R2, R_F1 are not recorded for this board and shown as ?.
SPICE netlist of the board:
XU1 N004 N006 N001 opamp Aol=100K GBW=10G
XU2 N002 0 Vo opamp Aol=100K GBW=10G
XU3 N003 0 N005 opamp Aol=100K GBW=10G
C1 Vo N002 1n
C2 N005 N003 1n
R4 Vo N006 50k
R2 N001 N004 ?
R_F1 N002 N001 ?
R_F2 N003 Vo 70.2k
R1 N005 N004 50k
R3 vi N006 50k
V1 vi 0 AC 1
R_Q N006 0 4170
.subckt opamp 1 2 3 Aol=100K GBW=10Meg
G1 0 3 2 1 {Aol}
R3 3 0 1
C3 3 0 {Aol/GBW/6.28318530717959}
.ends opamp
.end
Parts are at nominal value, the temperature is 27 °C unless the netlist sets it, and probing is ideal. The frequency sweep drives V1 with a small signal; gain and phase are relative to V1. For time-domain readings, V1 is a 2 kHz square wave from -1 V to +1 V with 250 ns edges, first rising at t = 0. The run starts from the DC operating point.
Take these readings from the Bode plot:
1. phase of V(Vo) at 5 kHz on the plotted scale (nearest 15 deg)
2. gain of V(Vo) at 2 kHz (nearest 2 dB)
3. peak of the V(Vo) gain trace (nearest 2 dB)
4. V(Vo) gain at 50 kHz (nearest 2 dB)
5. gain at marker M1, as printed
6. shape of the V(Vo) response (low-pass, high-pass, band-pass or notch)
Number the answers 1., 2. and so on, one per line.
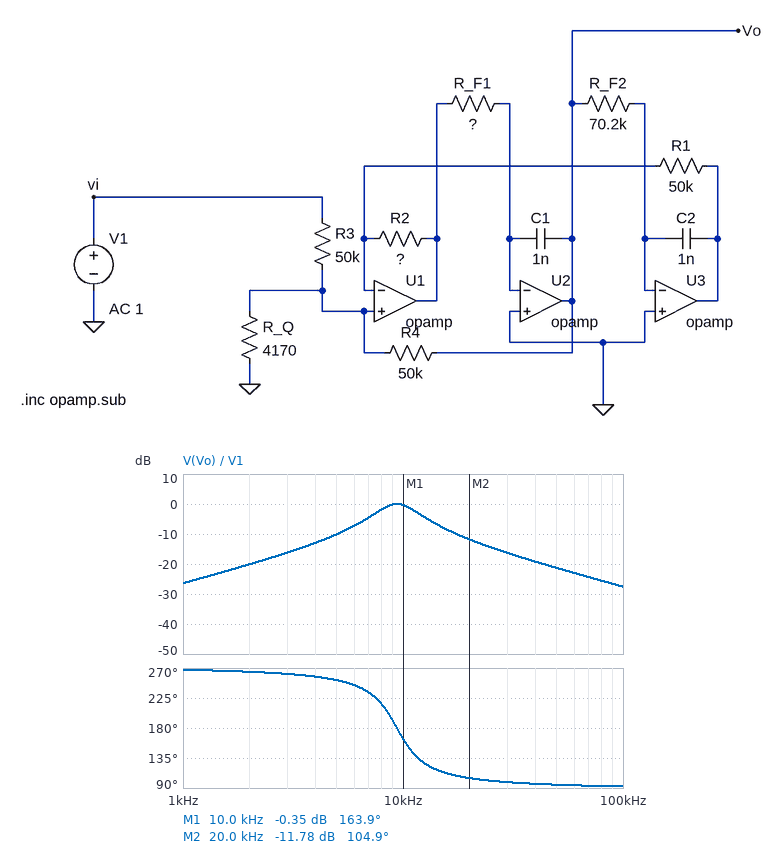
1. 255 deg
2. -20 dB
3. 0 dB
4. -22 dB
5. -0.35 dB
6. band-pass
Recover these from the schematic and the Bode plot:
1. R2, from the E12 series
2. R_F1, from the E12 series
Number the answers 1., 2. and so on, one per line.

1. 100 kΩ
2. 8.2 kΩ
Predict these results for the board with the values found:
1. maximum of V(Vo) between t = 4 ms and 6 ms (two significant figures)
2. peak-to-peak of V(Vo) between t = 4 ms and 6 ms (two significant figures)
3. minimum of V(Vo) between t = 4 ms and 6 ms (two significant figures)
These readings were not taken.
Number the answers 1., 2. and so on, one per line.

1. 650 mV
2. 1.3 V
3. -650 mV
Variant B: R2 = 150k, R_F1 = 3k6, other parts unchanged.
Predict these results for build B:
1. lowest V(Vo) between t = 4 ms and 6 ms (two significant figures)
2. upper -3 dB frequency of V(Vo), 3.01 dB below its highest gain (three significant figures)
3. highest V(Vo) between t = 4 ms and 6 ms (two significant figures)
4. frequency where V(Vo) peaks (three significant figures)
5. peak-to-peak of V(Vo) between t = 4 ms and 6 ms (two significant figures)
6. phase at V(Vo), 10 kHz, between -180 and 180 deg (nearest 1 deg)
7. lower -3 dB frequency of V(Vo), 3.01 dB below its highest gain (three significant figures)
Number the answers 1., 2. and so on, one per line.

1. -910 mV
2. 24.8 kHz
3. 910 mV
4. 17.3 kHz
5. 1.8 V
6. -122 deg
7. 12.1 kHz
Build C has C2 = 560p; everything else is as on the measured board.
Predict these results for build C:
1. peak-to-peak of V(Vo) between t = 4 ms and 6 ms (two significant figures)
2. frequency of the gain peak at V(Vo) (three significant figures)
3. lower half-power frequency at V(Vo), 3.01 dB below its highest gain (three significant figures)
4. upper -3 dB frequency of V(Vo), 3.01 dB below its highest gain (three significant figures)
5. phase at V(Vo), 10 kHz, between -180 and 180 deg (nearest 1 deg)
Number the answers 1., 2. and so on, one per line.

1. 1.0 V
2. 12.5 kHz
3. 10.6 kHz
4. 14.8 kHz
5. -126 deg
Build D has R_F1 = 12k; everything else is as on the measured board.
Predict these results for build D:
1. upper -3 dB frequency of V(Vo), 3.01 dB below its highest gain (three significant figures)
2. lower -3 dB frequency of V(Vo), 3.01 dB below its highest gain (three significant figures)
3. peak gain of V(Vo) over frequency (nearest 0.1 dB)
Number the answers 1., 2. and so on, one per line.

1. 9.31 kHz
2. 6.46 kHz
3. 0 dB
